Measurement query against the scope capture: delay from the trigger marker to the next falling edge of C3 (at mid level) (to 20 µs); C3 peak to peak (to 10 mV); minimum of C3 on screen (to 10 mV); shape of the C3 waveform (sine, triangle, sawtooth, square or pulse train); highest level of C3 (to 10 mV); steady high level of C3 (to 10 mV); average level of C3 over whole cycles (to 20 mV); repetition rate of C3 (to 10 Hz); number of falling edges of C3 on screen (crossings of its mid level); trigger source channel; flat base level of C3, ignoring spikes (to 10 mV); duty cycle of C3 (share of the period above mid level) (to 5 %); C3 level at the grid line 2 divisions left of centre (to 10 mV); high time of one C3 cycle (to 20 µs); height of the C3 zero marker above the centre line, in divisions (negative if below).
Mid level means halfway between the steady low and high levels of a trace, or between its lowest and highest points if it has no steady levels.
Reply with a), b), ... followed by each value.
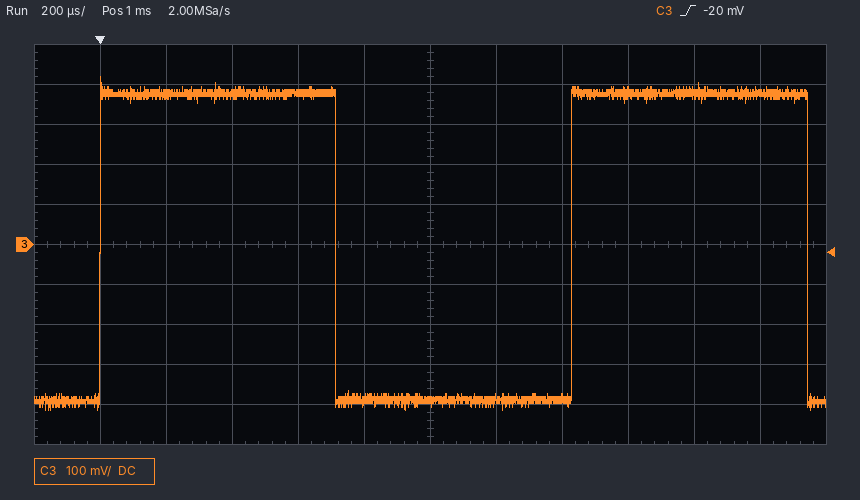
a) 720 µs
b) 830 mV
c) -410 mV
d) square
e) 420 mV
f) 380 mV
g) 0 mV
h) 700 Hz
i) 2
j) C3
k) -390 mV
l) 50 %
m) 380 mV
n) 720 µs
o) 0.0 div
